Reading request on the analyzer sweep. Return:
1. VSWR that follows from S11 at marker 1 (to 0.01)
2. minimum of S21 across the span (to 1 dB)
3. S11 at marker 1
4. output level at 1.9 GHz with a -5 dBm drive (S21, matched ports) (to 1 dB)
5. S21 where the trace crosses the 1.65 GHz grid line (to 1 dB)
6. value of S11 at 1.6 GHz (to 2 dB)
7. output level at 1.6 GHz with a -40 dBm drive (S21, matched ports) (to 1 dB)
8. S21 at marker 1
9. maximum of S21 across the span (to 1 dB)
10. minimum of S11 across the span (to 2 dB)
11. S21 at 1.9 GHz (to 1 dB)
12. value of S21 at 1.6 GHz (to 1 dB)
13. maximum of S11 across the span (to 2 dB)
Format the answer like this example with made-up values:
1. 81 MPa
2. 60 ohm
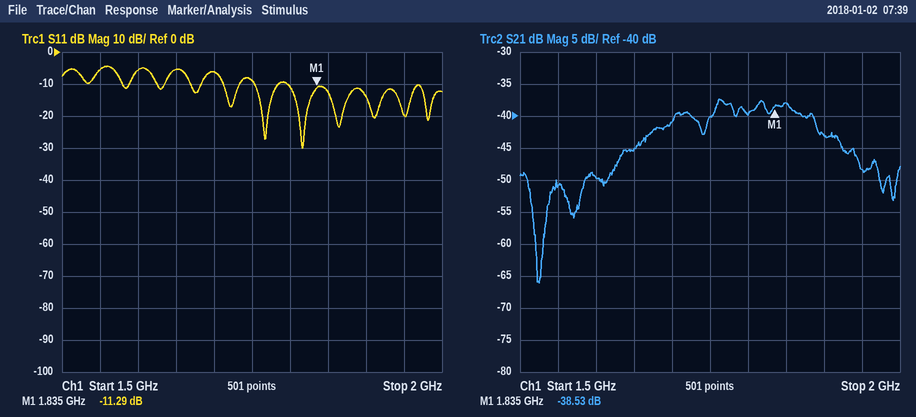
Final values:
1. 1.75
2. -66 dB
3. -11.29 dB
4. -48 dBm
5. -45 dB
6. -6 dB
7. -90 dBm
8. -38.53 dB
9. -37 dB
10. -30 dB
11. -43 dB
12. -50 dB
13. -4 dB
